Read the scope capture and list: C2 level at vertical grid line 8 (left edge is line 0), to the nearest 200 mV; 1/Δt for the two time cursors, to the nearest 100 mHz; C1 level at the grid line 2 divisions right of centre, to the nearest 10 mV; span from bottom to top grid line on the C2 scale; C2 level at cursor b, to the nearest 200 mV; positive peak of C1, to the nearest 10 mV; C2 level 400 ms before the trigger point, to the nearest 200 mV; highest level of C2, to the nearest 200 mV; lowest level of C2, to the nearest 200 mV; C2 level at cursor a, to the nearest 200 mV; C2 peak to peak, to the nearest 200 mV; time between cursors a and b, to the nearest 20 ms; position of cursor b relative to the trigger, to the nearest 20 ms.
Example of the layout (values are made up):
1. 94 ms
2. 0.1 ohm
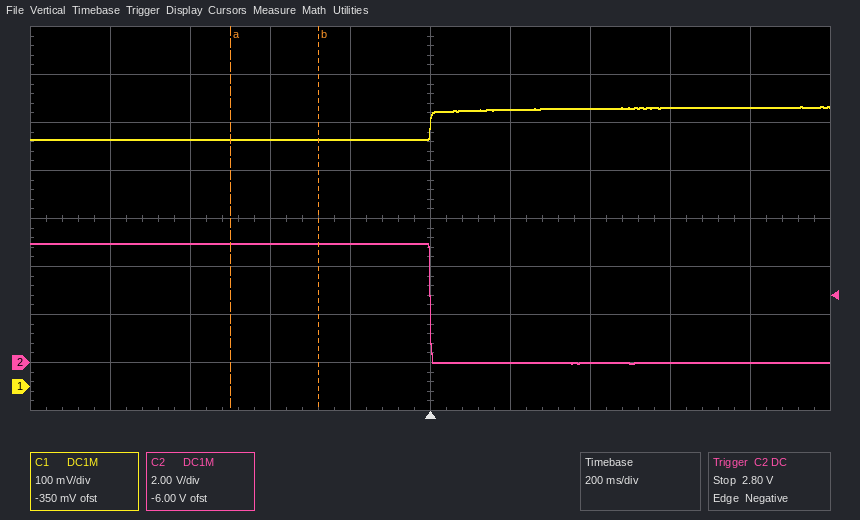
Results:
1. 0.0 V
2. 4.5 Hz
3. 580 mV
4. 16 V
5. 5.0 V
6. 580 mV
7. 5.0 V
8. 5.0 V
9. 0.0 V
10. 5.0 V
11. 5.0 V
12. 220 ms
13. -280 ms
